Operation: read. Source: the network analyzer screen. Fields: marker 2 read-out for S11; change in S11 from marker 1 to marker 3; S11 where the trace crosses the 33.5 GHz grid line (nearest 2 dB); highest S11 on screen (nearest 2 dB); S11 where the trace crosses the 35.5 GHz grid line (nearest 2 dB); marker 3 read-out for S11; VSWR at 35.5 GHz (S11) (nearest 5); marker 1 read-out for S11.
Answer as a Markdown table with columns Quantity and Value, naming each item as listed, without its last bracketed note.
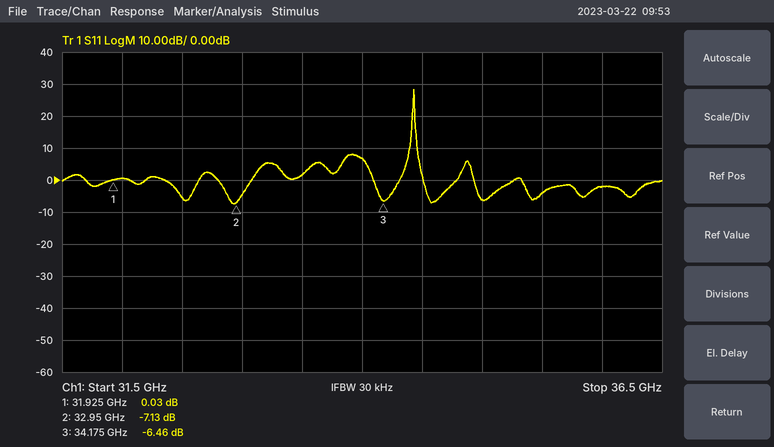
| Quantity | Value |
|---|---|
| marker 2 read-out for S11 | -7.13 dB |
| change in S11 from marker 1 to marker 3 | -6.49 dB |
| S11 where the trace crosses the 33.5 GHz grid line | 2 dB |
| highest S11 on screen | 28 dB |
| S11 where the trace crosses the 35.5 GHz grid line | -4 dB |
| marker 3 read-out for S11 | -6.46 dB |
| VSWR at 35.5 GHz (S11) | 5 |
| marker 1 read-out for S11 | 0.03 dB |
